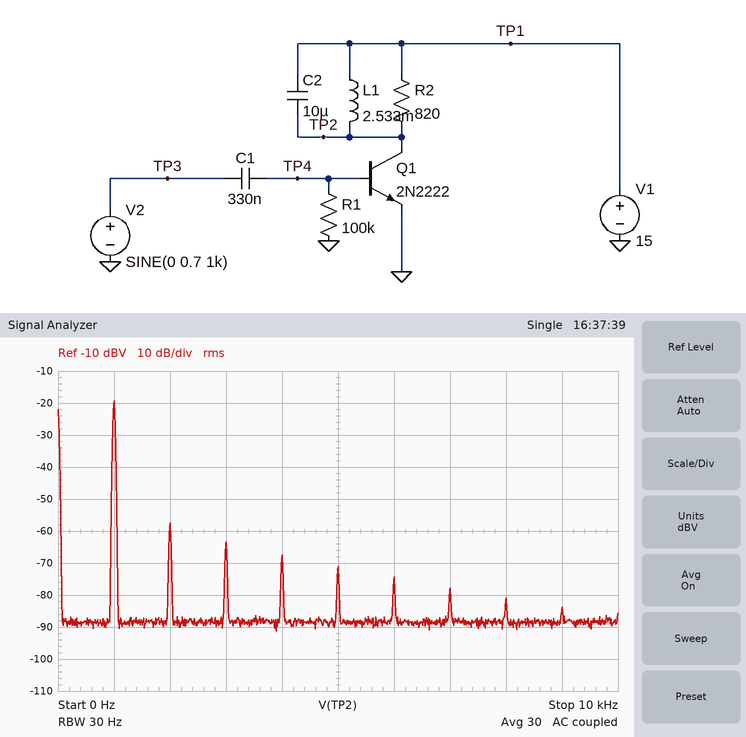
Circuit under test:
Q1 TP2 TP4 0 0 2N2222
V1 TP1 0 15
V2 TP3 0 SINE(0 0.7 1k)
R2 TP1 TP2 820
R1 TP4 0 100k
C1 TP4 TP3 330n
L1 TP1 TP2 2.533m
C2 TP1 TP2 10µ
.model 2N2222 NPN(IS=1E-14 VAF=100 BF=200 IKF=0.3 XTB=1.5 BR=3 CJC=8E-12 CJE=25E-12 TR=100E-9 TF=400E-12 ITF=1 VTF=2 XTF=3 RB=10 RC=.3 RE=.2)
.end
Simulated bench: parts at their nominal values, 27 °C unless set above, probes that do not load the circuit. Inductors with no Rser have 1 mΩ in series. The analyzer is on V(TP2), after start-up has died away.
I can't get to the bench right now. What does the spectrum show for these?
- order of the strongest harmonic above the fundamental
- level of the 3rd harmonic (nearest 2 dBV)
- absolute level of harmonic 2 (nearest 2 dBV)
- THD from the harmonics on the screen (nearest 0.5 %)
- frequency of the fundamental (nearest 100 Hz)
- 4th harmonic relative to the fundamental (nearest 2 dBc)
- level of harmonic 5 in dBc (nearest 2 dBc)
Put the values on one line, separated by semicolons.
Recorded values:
2; -64 dBV; -58 dBV; 1.5 %; 1.0 kHz; -48 dBc; -52 dBc
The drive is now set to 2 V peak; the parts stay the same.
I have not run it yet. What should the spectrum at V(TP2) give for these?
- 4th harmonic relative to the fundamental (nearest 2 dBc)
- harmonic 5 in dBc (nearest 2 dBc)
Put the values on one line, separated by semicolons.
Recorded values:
-46 dBc; -50 dBc
